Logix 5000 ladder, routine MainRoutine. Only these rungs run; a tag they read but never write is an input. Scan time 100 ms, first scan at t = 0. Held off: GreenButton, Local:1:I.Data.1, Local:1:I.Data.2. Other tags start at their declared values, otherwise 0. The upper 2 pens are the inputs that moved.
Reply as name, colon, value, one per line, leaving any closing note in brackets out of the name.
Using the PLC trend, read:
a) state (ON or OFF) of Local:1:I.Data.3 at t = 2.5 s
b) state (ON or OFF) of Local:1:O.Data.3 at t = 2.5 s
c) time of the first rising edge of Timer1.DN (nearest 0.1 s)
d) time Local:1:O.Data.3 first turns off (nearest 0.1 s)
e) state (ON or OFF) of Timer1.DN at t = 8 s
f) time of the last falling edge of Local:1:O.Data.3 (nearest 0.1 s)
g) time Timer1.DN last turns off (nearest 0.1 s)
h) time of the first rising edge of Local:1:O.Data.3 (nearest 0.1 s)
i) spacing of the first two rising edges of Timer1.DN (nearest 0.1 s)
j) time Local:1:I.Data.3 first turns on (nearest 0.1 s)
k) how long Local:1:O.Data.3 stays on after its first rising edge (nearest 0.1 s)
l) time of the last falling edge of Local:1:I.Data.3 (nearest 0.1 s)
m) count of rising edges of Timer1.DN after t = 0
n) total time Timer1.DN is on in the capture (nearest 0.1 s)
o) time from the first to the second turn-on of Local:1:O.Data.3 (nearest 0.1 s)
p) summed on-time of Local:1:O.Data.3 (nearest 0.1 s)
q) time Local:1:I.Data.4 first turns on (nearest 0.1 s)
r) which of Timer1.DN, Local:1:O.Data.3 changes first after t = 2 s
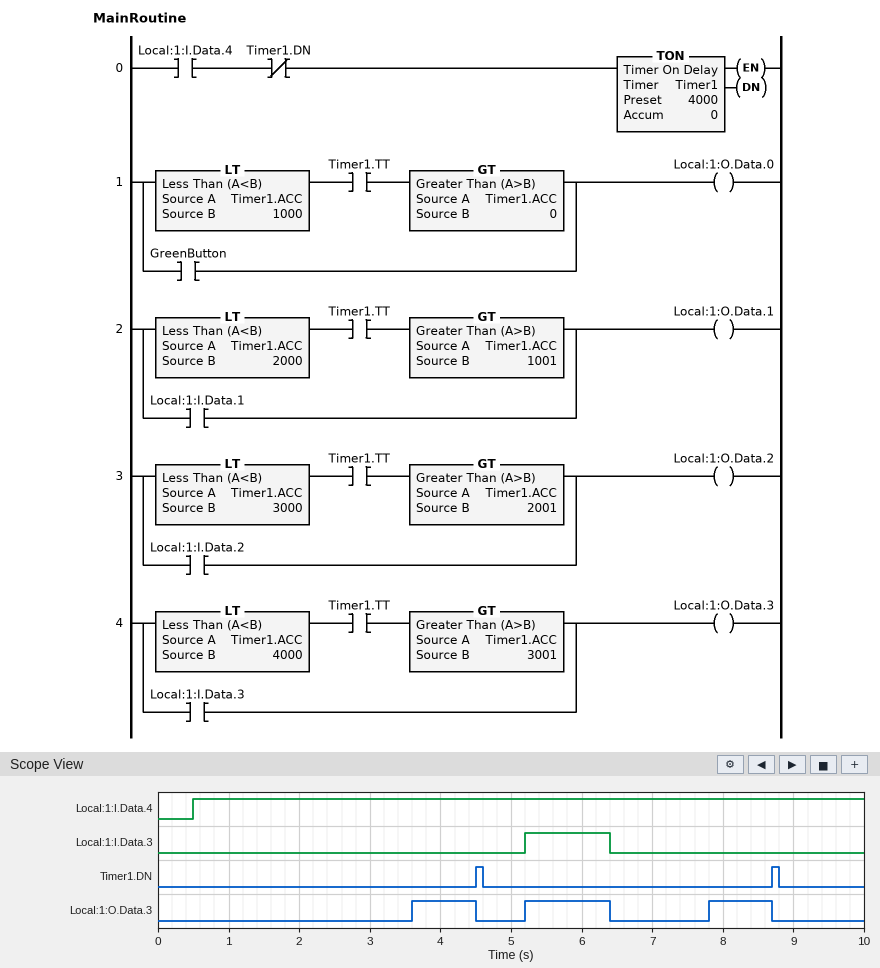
state (ON or OFF) of Local:1:I.Data.3 at t = 2.5 s: OFF
state (ON or OFF) of Local:1:O.Data.3 at t = 2.5 s: OFF
time of the first rising edge of Timer1.DN: 4.5 s
time Local:1:O.Data.3 first turns off: 4.5 s
state (ON or OFF) of Timer1.DN at t = 8 s: OFF
time of the last falling edge of Local:1:O.Data.3: 8.7 s
time Timer1.DN last turns off: 8.8 s
time of the first rising edge of Local:1:O.Data.3: 3.6 s
spacing of the first two rising edges of Timer1.DN: 4.2 s
time Local:1:I.Data.3 first turns on: 5.2 s
how long Local:1:O.Data.3 stays on after its first rising edge: 0.9 s
time of the last falling edge of Local:1:I.Data.3: 6.4 s
count of rising edges of Timer1.DN after t = 0: 2
total time Timer1.DN is on in the capture: 0.2 s
time from the first to the second turn-on of Local:1:O.Data.3: 1.6 s
summed on-time of Local:1:O.Data.3: 3.0 s
time Local:1:I.Data.4 first turns on: 0.5 s
which of Timer1.DN, Local:1:O.Data.3 changes first after t = 2 s: Local:1:O.Data.3
